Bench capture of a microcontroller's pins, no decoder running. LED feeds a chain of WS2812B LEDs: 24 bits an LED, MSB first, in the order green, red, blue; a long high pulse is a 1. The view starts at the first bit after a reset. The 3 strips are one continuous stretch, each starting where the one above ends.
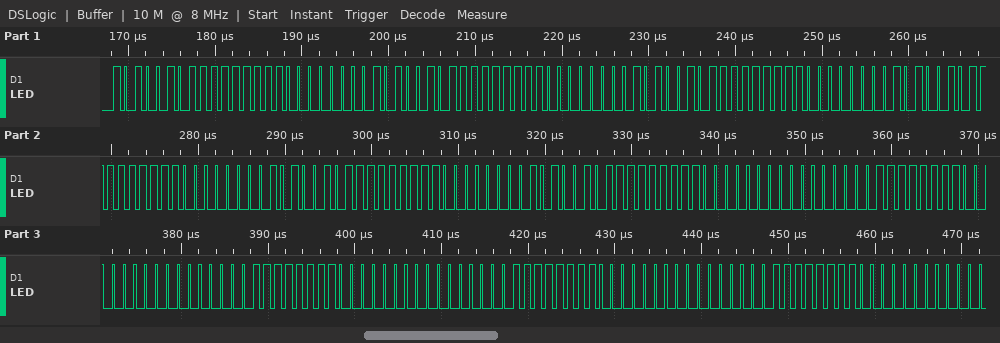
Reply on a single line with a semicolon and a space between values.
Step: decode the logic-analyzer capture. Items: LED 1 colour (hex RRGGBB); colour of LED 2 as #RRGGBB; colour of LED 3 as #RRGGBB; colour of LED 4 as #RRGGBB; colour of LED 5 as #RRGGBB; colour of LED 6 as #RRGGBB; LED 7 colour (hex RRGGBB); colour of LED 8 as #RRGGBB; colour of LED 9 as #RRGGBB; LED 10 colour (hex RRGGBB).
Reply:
#FFA500; #FFA500; #FFA500; #FFA500; #FFA500; #FFA500; #FF0000; #FF0000; #FF0000; #FF0000
